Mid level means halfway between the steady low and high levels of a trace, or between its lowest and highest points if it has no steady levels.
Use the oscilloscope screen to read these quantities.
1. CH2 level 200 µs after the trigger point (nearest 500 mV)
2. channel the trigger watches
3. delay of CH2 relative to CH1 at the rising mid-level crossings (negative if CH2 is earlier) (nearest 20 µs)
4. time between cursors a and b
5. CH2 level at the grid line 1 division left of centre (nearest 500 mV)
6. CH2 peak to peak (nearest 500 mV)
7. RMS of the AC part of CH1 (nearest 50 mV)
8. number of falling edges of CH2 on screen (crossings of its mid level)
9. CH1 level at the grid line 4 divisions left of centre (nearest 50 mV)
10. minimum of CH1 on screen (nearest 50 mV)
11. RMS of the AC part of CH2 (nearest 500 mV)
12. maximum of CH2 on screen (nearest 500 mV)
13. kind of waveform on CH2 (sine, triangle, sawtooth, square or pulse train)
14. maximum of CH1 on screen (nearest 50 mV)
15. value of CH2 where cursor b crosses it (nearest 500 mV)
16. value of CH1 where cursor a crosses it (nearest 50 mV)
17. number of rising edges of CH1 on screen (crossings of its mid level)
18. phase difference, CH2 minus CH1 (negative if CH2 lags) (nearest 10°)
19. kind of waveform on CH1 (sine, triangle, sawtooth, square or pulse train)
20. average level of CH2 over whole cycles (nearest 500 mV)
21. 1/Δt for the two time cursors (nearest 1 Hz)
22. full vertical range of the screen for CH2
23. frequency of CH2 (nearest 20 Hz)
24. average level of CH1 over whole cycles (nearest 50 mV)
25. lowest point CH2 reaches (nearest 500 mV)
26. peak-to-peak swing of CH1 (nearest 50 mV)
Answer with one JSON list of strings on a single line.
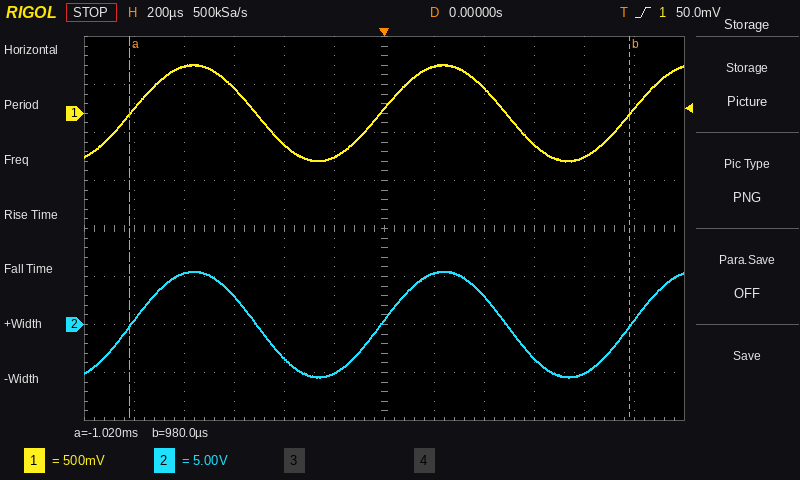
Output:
["5.5 V", "CH1", "0 µs", "2.00 ms", "-5.0 V", "11.0 V", "350 mV", "2", "500 mV", "-500 mV", "4.0 V", "5.5 V", "sine", "500 mV", "0.0 V", "0 mV", "3", "0°", "sine", "0.0 V", "500 Hz", "40 V", "1.00 kHz", "0 mV", "-5.5 V", "1.00 V"]
